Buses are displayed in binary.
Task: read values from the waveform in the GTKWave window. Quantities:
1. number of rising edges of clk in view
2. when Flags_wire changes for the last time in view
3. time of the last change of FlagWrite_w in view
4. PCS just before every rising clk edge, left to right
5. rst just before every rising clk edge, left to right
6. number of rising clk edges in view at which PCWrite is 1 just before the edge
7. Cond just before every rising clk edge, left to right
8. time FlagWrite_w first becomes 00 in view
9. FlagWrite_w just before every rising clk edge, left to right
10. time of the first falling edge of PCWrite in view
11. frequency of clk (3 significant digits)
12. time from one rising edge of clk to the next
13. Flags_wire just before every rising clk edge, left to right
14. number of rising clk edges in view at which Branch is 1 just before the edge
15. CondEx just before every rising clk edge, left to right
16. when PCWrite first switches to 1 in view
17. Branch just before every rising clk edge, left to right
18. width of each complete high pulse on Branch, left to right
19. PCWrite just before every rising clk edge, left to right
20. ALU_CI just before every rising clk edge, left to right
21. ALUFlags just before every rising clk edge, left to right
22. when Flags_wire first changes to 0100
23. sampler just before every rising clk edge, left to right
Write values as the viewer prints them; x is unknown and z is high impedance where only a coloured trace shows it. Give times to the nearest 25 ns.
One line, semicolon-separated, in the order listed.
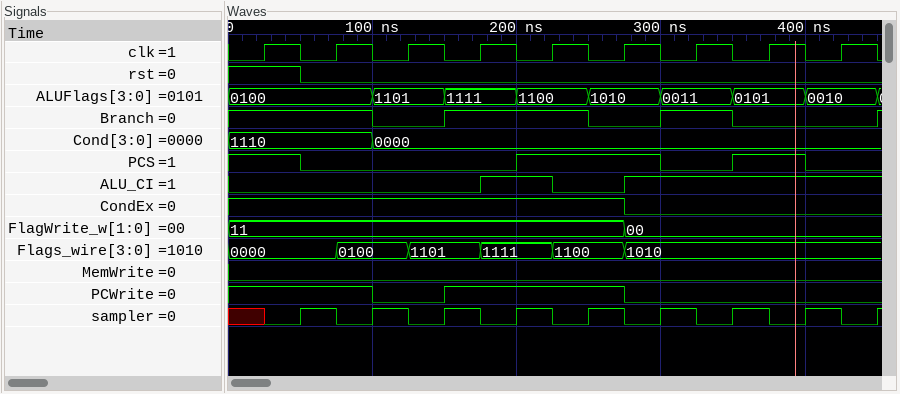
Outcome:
9; 275 ns; 275 ns; 1 0 0 0 1 1 0 1 0; 1 0 0 0 0 0 0 0 0; 5; 1110, 1110, 0000, 0000, 0000, 0000, 0000, 0000, 0000; 275 ns; 11, 11, 11, 11, 11, 11, 00, 00, 00; 100 ns; 20.0 MHz; 50 ns; 0000, 0000, 0100, 1101, 1111, 1100, 1010, 1010, 1010; 5; 1 1 1 1 1 1 0 0 0; 150 ns; 1 1 0 1 1 0 1 0 0; 100 ns, 50 ns; 1 1 0 1 1 1 0 0 0; 0 0 0 0 1 0 1 1 1; 0100, 0100, 1101, 1111, 1100, 1010, 0011, 0101, 0010; 75 ns; x 1 1 1 1 1 1 1 1
